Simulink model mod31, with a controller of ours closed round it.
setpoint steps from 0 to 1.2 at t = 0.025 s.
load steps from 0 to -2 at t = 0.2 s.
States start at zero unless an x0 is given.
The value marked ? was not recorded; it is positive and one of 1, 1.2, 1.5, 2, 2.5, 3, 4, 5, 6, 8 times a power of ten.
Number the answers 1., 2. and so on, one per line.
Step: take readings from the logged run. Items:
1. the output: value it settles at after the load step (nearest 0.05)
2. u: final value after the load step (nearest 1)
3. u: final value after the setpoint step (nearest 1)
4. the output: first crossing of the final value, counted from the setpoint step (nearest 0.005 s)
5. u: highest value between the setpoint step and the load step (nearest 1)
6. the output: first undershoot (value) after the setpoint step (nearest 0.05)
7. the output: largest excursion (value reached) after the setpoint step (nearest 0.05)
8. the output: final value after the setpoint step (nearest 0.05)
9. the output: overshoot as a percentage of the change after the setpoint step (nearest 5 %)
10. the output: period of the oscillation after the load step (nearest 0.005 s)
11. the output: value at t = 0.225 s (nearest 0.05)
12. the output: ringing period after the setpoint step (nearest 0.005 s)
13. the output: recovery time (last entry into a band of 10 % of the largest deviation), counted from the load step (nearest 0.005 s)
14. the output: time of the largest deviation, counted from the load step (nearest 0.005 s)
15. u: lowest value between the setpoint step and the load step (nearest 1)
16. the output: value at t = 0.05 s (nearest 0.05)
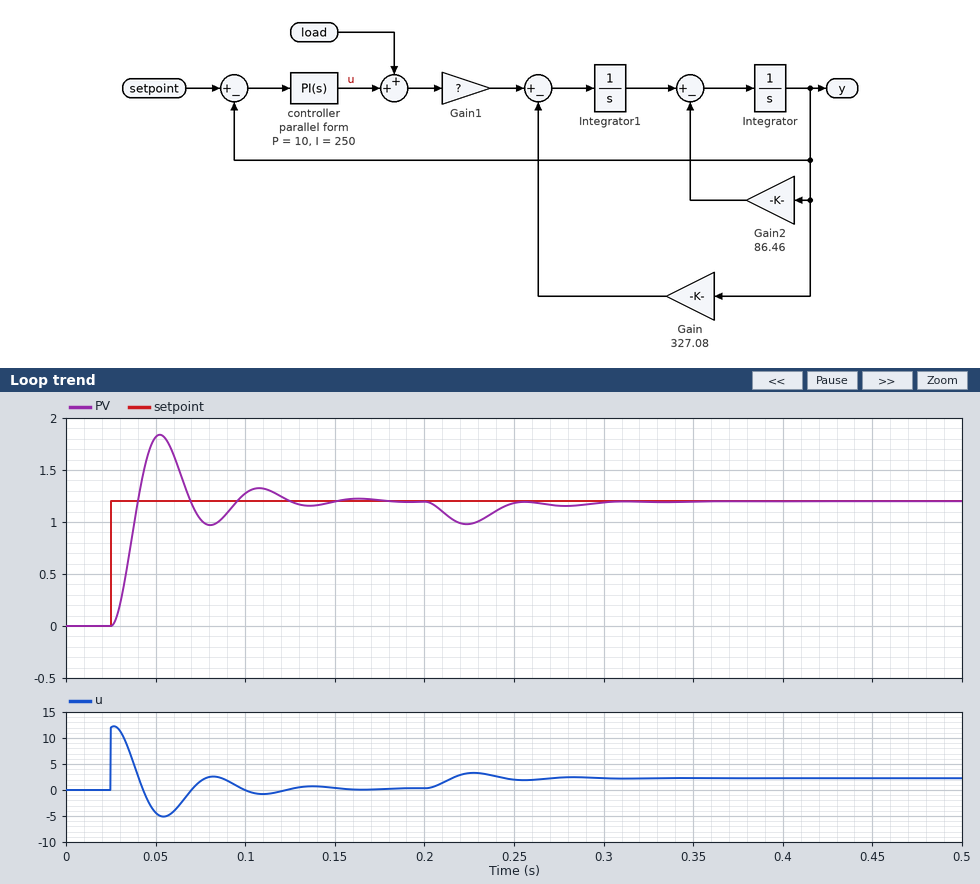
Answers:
1. 1.20
2. 2
3. 0
4. 0.015 s
5. 12
6. 0.95
7. 1.85
8. 1.20
9. 55 %
10. 0.055 s
11. 1.00
12. 0.055 s
13. 0.095 s
14. 0.025 s
15. -5
16. 1.80
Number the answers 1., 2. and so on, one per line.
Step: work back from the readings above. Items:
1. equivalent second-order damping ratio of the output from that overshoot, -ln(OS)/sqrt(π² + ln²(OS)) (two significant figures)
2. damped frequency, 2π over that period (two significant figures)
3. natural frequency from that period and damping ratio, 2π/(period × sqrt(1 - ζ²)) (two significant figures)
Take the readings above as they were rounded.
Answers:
1. 0.19
2. 110 rad/s
3. 120 rad/s
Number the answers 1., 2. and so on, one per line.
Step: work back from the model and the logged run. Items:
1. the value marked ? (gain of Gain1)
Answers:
1. 1500
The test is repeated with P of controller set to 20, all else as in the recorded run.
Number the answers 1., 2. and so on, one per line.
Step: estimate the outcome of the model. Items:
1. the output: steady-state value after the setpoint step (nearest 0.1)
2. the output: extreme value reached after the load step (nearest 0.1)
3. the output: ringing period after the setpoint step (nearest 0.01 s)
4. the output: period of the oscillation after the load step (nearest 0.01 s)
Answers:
1. 1.2
2. 1.1
3. 0.04 s
4. 0.04 s
